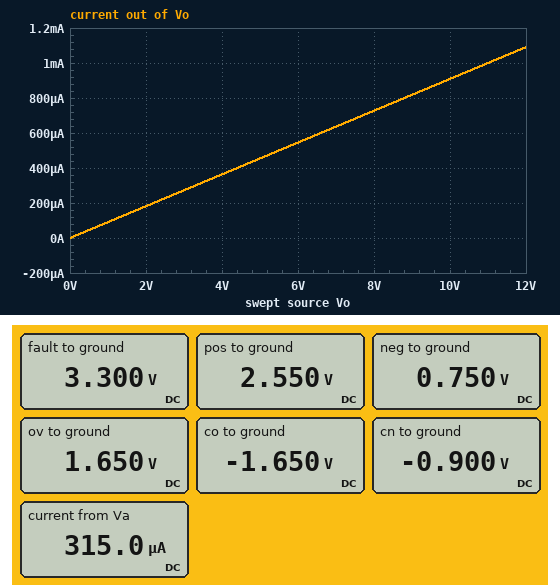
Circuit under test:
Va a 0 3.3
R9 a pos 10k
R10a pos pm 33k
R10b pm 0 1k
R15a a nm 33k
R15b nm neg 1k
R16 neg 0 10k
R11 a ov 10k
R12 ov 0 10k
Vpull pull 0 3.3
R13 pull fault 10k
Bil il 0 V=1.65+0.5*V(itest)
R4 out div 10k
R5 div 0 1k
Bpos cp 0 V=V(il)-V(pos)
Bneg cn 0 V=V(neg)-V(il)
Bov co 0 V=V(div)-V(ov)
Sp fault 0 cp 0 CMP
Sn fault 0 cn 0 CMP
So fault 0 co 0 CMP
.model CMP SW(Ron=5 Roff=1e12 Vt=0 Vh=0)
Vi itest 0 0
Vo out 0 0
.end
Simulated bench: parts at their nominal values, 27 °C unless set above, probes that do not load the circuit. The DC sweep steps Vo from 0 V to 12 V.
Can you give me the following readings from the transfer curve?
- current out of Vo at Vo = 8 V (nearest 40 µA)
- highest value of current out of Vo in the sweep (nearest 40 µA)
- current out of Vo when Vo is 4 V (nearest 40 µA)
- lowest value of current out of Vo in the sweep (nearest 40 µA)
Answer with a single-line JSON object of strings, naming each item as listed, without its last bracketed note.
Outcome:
{"current out of Vo at Vo = 8 V": "720 µA", "highest value of current out of Vo in the sweep": "1.08 mA", "current out of Vo when Vo is 4 V": "360 µA", "lowest value of current out of Vo in the sweep": "0 A"}
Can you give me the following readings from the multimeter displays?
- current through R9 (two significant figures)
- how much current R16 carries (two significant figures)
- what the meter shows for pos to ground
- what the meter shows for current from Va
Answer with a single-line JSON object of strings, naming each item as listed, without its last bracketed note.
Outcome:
{"current through R9": "75 µA", "how much current R16 carries": "75 µA", "what the meter shows for pos to ground": "2.550 V", "what the meter shows for current from Va": "315.0 µA"}
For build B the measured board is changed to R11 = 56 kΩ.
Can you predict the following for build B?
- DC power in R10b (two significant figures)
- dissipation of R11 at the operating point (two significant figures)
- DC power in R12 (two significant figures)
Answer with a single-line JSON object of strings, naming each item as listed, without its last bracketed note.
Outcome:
{"DC power in R10b": "5.6 µW", "dissipation of R11 at the operating point": "140 µW", "DC power in R12": "25 µW"}
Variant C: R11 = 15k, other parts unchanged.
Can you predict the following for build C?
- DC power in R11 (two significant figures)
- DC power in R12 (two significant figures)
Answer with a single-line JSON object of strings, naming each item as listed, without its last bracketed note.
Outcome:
{"DC power in R11": "260 µW", "DC power in R12": "170 µW"}
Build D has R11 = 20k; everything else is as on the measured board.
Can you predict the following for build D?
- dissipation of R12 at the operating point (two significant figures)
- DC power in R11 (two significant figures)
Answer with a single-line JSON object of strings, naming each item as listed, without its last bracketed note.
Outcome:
{"dissipation of R12 at the operating point": "120 µW", "DC power in R11": "240 µW"}
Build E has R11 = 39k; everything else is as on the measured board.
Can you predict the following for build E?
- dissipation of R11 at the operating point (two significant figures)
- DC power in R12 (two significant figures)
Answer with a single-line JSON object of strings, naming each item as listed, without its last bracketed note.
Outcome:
{"dissipation of R11 at the operating point": "180 µW", "DC power in R12": "45 µW"}
